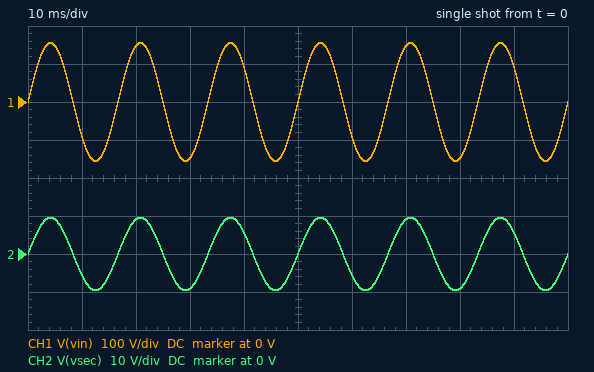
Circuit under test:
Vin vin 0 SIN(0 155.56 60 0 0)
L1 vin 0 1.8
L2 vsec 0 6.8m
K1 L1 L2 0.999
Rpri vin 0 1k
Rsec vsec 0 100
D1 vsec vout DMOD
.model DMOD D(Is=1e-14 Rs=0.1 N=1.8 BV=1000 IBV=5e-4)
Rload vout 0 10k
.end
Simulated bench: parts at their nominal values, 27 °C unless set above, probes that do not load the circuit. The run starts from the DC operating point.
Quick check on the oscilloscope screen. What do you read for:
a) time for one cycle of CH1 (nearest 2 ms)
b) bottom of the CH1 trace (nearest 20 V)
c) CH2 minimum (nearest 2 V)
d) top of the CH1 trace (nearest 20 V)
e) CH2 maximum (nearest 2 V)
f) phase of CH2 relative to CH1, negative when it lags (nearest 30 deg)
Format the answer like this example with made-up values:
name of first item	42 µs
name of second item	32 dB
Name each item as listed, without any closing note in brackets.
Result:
time for one cycle of CH1	16 ms
bottom of the CH1 trace	-160 V
CH2 minimum	-10 V
top of the CH1 trace	160 V
CH2 maximum	10 V
phase of CH2 relative to CH1, negative when it lags	0 deg
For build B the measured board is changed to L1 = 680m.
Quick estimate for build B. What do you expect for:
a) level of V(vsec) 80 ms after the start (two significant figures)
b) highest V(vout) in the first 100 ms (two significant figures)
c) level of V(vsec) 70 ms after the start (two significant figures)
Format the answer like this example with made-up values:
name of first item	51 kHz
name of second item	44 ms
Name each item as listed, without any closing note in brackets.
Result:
level of V(vsec) 80 ms after the start	-15 V
highest V(vout) in the first 100 ms	14 V
level of V(vsec) 70 ms after the start	15 V
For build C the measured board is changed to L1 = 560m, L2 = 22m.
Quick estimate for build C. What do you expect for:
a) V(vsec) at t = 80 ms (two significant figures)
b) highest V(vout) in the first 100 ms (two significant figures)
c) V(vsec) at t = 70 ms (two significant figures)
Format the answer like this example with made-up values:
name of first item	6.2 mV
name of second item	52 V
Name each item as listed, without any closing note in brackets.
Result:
V(vsec) at t = 80 ms	-29 V
highest V(vout) in the first 100 ms	30 V
V(vsec) at t = 70 ms	29 V
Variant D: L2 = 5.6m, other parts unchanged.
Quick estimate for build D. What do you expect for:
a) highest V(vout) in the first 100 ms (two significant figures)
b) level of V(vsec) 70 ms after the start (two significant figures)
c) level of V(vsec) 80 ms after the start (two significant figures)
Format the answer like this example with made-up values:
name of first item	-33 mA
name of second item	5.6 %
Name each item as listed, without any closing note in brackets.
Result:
highest V(vout) in the first 100 ms	7.5 V
level of V(vsec) 70 ms after the start	8.2 V
level of V(vsec) 80 ms after the start	-8.2 V
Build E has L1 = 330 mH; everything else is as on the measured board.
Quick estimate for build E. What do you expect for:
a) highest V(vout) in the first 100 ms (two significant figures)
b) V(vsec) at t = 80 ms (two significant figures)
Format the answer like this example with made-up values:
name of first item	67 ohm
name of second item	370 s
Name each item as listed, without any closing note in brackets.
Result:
highest V(vout) in the first 100 ms	21 V
V(vsec) at t = 80 ms	-21 V
